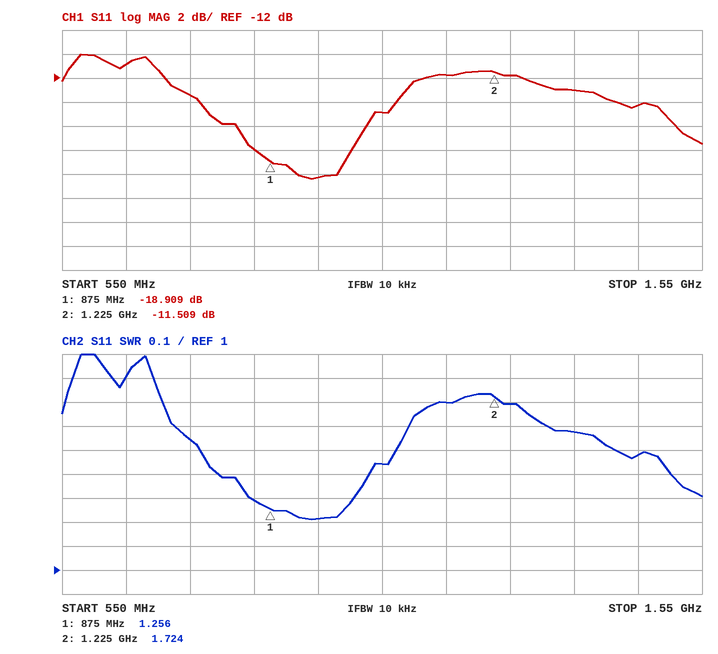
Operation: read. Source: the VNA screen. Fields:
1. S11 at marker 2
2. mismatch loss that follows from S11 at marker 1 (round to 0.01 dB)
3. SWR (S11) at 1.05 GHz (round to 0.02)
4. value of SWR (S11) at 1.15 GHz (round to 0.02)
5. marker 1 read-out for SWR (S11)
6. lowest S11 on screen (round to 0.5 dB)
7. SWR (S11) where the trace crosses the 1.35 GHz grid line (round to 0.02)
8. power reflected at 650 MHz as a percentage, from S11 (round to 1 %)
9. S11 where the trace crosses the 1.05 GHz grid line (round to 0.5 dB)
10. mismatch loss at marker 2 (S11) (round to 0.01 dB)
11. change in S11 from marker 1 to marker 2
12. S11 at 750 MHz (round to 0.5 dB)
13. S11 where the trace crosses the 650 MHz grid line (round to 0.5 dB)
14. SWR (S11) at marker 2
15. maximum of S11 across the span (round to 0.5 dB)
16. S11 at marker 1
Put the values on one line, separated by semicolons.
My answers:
-11.509 dB; 0.06 dB; 1.44; 1.70; 1.256; -20.5 dB; 1.58; 8 %; -15.0 dB; 0.32 dB; 7.400 dB; -13.5 dB; -11.0 dB; 1.724; -10.0 dB; -18.909 dB
